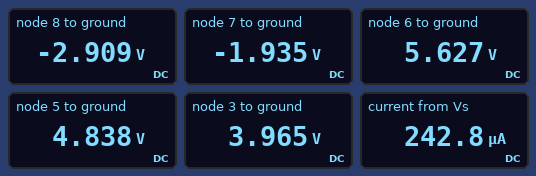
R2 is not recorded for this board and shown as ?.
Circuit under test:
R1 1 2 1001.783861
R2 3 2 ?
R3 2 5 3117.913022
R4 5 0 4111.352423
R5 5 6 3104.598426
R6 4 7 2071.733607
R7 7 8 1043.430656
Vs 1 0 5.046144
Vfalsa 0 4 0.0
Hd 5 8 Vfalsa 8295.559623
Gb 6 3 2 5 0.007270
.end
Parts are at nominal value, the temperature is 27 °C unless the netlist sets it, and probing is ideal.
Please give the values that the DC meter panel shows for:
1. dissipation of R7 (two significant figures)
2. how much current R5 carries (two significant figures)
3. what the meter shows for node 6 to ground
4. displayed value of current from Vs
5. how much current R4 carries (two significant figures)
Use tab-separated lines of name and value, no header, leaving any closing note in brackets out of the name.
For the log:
dissipation of R7	910 µW
how much current R5 carries	250 µA
what the meter shows for node 6 to ground	5.627 V
displayed value of current from Vs	242.8 µA
how much current R4 carries	1.2 mA
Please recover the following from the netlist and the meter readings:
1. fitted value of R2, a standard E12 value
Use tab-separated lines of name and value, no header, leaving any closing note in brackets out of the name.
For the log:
fitted value of R2, a standard E12 value	3.3 kΩ
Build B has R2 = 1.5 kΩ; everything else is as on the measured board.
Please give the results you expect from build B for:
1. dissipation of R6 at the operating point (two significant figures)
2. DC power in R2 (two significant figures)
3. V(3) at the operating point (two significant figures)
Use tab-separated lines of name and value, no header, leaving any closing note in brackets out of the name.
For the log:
dissipation of R6 at the operating point	1.8 mW
DC power in R2	97 µW
V(3) at the operating point	4.4 V
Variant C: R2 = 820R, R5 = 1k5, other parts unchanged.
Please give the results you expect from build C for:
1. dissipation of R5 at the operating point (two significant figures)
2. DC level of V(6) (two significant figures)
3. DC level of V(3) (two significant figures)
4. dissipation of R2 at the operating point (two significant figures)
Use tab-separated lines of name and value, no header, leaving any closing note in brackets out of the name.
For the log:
dissipation of R5 at the operating point	97 µW
DC level of V(6)	5.2 V
DC level of V(3)	4.6 V
dissipation of R2 at the operating point	53 µW
